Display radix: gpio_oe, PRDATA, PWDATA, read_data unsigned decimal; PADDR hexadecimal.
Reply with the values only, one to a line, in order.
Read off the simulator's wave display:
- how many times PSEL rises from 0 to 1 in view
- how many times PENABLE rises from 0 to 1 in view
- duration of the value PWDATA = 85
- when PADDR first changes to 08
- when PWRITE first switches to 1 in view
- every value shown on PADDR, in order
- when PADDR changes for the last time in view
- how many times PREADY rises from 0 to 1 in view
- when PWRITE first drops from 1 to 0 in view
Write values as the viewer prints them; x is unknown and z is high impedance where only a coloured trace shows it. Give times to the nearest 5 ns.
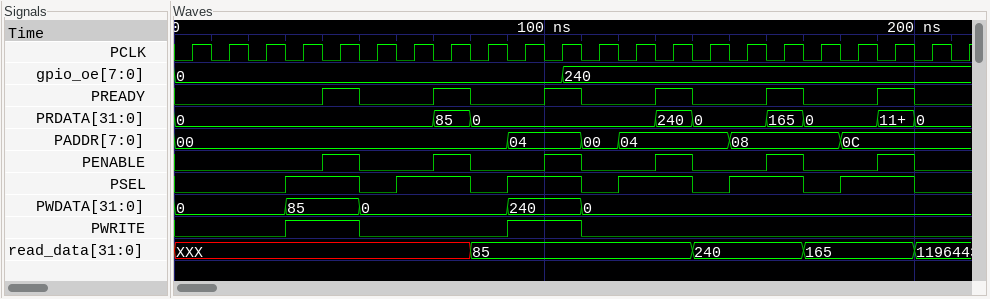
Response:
6
6
20 ns
150 ns
30 ns
00, 04, 00, 04, 08, 0C
180 ns
6
50 ns
